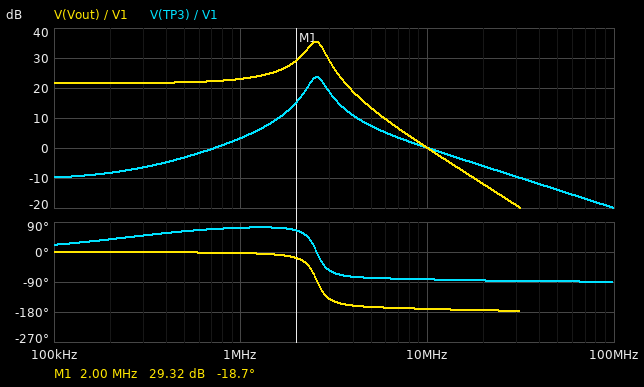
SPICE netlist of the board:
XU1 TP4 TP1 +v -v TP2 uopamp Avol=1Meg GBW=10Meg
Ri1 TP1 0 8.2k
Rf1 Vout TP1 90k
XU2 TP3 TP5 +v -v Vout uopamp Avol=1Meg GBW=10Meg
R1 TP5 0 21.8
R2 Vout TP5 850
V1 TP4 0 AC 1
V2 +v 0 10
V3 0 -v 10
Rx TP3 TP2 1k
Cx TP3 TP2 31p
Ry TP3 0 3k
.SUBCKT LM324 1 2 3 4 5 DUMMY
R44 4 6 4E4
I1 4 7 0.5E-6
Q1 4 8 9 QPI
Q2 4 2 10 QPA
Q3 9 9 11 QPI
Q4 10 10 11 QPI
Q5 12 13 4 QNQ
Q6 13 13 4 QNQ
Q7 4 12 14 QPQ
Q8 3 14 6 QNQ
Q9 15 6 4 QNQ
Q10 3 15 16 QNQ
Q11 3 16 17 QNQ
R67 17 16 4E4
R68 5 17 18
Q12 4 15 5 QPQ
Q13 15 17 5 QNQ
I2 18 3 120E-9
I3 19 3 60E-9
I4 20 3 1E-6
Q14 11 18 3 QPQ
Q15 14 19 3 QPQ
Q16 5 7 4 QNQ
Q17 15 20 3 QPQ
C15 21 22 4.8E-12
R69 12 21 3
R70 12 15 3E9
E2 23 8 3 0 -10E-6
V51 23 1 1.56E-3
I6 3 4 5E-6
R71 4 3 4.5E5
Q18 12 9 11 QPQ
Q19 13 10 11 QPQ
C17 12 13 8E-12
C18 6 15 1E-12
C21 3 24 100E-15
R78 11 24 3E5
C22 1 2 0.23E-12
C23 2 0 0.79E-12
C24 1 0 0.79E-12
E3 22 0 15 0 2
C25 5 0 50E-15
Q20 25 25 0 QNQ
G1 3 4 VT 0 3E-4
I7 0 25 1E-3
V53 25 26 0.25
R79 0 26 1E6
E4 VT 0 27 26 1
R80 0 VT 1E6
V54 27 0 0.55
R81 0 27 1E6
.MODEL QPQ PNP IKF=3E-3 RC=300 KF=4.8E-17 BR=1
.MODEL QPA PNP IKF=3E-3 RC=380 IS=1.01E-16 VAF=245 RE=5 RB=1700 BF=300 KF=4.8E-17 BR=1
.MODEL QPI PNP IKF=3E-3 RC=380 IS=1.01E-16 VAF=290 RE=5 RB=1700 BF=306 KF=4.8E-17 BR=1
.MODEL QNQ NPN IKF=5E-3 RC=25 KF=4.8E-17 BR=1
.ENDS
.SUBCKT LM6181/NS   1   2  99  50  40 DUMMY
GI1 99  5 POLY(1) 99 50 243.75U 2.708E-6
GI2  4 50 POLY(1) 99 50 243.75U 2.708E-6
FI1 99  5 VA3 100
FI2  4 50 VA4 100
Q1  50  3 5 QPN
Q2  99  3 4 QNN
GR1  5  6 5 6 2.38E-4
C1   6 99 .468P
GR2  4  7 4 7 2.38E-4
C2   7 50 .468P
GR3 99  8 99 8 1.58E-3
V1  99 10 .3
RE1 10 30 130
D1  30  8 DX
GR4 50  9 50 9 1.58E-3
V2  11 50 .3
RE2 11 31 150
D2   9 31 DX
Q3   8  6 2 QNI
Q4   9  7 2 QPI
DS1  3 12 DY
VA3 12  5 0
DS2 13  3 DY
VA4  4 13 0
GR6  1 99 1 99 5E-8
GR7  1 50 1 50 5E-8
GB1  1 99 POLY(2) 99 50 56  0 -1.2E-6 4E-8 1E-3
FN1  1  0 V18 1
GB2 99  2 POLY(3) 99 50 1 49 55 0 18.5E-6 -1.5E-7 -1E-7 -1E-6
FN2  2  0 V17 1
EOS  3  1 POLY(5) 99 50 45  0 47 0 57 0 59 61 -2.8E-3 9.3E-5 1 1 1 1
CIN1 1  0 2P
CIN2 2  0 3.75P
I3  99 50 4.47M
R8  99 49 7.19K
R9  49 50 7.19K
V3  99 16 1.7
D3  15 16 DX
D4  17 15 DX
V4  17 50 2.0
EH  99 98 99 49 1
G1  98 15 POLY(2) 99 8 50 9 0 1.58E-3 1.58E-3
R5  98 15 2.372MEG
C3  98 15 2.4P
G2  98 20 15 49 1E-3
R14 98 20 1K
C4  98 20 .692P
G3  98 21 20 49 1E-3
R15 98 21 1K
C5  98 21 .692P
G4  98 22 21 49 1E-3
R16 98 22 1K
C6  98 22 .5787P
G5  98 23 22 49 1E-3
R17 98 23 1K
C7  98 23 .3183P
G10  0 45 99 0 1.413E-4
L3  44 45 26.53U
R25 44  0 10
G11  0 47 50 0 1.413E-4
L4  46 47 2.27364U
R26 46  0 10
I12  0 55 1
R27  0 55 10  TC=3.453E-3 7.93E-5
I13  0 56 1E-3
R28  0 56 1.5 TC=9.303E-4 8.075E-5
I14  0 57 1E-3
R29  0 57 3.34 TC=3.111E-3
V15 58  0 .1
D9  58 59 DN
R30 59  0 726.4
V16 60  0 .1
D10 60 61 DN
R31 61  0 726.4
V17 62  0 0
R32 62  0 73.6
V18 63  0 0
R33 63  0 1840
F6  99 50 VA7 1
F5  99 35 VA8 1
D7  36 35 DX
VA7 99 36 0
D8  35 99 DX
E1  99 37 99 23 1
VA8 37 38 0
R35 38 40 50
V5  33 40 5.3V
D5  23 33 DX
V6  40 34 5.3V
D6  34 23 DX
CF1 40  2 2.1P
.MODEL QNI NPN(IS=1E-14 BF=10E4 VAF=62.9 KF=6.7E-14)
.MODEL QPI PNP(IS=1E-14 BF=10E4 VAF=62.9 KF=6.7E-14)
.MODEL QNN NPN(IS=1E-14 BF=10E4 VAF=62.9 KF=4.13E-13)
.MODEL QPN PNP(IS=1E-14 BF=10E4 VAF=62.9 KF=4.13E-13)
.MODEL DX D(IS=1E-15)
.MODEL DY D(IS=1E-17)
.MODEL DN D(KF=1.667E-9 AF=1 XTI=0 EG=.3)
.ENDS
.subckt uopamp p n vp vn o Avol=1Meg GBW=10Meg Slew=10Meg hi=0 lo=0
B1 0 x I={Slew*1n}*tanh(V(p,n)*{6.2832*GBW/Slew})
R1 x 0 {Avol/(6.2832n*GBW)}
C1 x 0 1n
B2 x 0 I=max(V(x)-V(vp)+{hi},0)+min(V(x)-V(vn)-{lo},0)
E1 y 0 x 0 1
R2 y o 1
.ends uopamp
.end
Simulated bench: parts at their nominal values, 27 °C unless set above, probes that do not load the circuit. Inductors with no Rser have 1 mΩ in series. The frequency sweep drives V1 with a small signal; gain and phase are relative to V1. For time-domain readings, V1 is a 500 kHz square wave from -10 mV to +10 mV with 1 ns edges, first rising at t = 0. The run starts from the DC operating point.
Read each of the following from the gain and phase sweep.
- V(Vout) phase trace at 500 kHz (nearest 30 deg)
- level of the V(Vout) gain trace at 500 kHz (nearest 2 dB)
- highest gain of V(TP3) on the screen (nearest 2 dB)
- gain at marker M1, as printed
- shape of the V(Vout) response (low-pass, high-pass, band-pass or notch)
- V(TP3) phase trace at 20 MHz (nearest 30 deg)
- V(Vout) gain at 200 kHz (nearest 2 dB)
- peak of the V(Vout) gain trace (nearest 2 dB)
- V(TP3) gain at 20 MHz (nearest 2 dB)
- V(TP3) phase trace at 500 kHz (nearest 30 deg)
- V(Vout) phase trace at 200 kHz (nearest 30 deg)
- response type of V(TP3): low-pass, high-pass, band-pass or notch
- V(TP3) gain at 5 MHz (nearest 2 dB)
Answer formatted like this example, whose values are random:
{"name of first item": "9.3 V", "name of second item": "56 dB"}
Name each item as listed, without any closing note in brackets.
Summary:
{"V(Vout) phase trace at 500 kHz": "0 deg", "level of the V(Vout) gain trace at 500 kHz": "22 dB", "highest gain of V(TP3) on the screen": "24 dB", "gain at marker M1, as printed": "29.32 dB", "shape of the V(Vout) response": "low-pass", "V(TP3) phase trace at 20 MHz": "-90 deg", "V(Vout) gain at 200 kHz": "22 dB", "peak of the V(Vout) gain trace": "36 dB", "V(TP3) gain at 20 MHz": "-6 dB", "V(TP3) phase trace at 500 kHz": "60 deg", "V(Vout) phase trace at 200 kHz": "0 deg", "response type of V(TP3): low-pass, high-pass, band-pass or notch": "band-pass", "V(TP3) gain at 5 MHz": "8 dB"}
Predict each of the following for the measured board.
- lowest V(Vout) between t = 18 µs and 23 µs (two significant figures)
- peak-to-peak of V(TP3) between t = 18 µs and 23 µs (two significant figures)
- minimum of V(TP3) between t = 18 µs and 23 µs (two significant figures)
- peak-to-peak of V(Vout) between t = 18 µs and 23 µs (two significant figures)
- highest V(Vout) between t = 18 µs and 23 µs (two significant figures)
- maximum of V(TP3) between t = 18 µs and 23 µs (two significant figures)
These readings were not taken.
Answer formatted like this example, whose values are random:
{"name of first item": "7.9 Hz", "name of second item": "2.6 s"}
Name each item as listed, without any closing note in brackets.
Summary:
{"lowest V(Vout) between t = 18 µs and 23 µs": "-340 mV", "peak-to-peak of V(TP3) between t = 18 µs and 23 µs": "140 mV", "minimum of V(TP3) between t = 18 µs and 23 µs": "-71 mV", "peak-to-peak of V(Vout) between t = 18 µs and 23 µs": "690 mV", "highest V(Vout) between t = 18 µs and 23 µs": "340 mV", "maximum of V(TP3) between t = 18 µs and 23 µs": "71 mV"}
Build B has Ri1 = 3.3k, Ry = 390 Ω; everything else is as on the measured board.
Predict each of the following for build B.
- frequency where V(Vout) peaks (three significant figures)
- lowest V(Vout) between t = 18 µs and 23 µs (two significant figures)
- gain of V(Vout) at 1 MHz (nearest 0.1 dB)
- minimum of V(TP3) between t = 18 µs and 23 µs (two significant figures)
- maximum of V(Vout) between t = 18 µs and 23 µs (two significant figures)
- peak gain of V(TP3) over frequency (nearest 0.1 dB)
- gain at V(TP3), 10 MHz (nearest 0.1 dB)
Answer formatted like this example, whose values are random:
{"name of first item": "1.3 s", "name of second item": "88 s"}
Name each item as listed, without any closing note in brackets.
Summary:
{"frequency where V(Vout) peaks": "961 kHz", "lowest V(Vout) between t = 18 µs and 23 µs": "-520 mV", "gain of V(Vout) at 1 MHz": "37.3 dB", "minimum of V(TP3) between t = 18 µs and 23 µs": "-39 mV", "maximum of V(Vout) between t = 18 µs and 23 µs": "520 mV", "peak gain of V(TP3) over frequency": "17.6 dB", "gain at V(TP3), 10 MHz": "-5.2 dB"}
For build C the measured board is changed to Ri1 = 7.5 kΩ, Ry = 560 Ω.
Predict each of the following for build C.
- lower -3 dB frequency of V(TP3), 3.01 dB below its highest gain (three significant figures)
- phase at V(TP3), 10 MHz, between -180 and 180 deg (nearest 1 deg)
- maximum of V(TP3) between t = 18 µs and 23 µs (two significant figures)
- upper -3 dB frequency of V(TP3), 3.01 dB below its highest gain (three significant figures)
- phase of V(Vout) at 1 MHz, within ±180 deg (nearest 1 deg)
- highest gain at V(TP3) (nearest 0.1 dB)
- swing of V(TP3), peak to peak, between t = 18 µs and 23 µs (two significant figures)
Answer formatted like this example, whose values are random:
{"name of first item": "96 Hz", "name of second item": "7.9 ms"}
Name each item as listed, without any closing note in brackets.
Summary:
{"lower -3 dB frequency of V(TP3), 3.01 dB below its highest gain": "1.41 MHz", "phase at V(TP3), 10 MHz, between -180 and 180 deg": "-61 deg", "maximum of V(TP3) between t = 18 µs and 23 µs": "42 mV", "upper -3 dB frequency of V(TP3), 3.01 dB below its highest gain": "2.02 MHz", "phase of V(Vout) at 1 MHz, within ±180 deg": "-11 deg", "highest gain at V(TP3)": "16.2 dB", "swing of V(TP3), peak to peak, between t = 18 µs and 23 µs": "83 mV"}
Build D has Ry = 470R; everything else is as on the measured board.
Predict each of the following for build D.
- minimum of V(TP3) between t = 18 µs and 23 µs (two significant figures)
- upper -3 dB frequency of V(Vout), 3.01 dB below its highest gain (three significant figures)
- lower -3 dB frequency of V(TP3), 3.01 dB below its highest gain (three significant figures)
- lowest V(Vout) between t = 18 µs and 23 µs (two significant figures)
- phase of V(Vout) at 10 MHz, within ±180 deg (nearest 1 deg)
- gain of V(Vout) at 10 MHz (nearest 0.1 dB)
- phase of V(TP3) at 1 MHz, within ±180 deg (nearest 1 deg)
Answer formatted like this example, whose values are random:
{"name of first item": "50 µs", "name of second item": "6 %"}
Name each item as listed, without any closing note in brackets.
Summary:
{"minimum of V(TP3) between t = 18 µs and 23 µs": "-38 mV", "upper -3 dB frequency of V(Vout), 3.01 dB below its highest gain": "1.89 MHz", "lower -3 dB frequency of V(TP3), 3.01 dB below its highest gain": "1.38 MHz", "lowest V(Vout) between t = 18 µs and 23 µs": "-280 mV", "phase of V(Vout) at 10 MHz, within ±180 deg": "-146 deg", "gain of V(Vout) at 10 MHz": "-4.2 dB", "phase of V(TP3) at 1 MHz, within ±180 deg": "64 deg"}
